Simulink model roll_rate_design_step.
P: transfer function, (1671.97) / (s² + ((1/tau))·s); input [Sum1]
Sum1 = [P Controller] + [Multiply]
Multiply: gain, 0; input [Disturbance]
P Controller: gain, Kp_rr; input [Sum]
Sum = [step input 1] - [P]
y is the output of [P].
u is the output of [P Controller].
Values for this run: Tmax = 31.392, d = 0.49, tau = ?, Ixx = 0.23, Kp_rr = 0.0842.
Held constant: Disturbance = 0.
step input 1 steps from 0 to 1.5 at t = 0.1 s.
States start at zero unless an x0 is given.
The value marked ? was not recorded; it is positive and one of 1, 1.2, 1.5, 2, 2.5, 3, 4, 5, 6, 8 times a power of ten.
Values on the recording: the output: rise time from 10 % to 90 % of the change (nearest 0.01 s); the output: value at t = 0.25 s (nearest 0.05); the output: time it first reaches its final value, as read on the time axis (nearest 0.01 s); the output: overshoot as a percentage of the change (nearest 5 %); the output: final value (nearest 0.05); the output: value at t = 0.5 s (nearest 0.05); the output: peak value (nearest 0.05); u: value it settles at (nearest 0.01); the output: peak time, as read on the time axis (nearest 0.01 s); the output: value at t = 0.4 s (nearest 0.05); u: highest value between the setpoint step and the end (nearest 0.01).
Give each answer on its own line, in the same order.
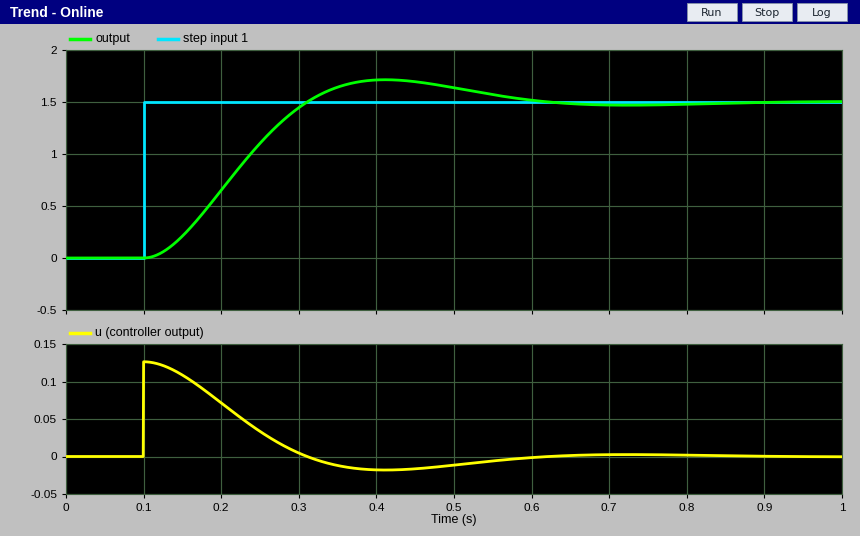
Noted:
0.14 s
1.10
0.31 s
15 %
1.50
1.65
1.70
0.00
0.41 s
1.70
0.13
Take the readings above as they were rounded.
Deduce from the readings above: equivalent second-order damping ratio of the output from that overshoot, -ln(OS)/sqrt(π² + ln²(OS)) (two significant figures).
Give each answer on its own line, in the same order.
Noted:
0.52
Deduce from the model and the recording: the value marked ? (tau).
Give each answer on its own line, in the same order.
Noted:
0.08
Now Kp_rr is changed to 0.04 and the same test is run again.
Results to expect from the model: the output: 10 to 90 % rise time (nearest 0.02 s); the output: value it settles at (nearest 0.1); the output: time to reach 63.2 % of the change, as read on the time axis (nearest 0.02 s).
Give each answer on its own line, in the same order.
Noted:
0.28 s
1.5
0.32 s
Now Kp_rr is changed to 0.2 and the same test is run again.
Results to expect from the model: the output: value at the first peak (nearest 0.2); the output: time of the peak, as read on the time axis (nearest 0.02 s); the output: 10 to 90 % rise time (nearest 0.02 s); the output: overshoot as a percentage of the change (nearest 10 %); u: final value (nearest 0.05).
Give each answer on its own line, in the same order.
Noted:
2.0
0.28 s
0.08 s
30 %
0.00
